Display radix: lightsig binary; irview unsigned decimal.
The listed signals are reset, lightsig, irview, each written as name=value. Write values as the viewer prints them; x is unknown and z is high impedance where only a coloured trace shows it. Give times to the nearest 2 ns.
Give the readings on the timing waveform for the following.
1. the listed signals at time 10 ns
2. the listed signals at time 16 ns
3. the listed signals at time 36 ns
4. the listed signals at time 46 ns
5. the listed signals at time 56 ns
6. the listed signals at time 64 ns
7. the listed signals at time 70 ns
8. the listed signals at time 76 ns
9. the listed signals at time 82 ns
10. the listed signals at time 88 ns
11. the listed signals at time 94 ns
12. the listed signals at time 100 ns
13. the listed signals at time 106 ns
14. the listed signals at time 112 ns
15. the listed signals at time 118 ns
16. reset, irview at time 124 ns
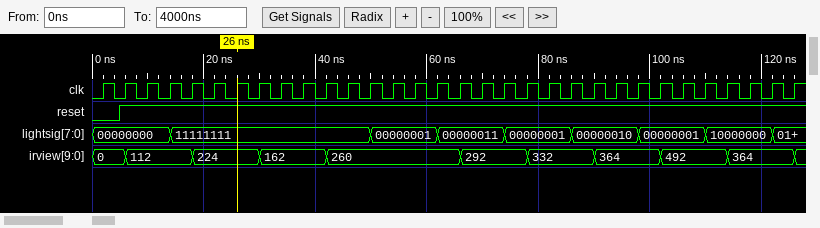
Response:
reset=1, lightsig=00000000, irview=112
reset=1, lightsig=11111111, irview=112
reset=1, lightsig=11111111, irview=162
reset=1, lightsig=11111111, irview=260
reset=1, lightsig=00000001, irview=260
reset=1, lightsig=00000011, irview=260
reset=1, lightsig=00000011, irview=292
reset=1, lightsig=00000001, irview=292
reset=1, lightsig=00000001, irview=332
reset=1, lightsig=00000010, irview=332
reset=1, lightsig=00000010, irview=364
reset=1, lightsig=00000001, irview=364
reset=1, lightsig=00000001, irview=492
reset=1, lightsig=10000000, irview=492
reset=1, lightsig=10000000, irview=364
reset=1, irview=364
